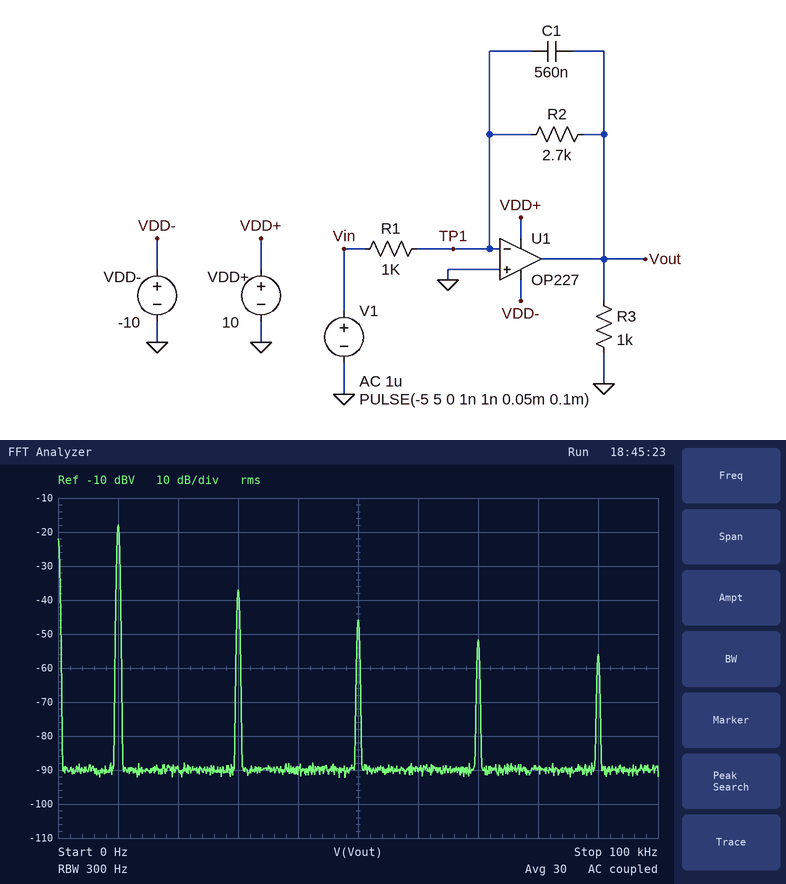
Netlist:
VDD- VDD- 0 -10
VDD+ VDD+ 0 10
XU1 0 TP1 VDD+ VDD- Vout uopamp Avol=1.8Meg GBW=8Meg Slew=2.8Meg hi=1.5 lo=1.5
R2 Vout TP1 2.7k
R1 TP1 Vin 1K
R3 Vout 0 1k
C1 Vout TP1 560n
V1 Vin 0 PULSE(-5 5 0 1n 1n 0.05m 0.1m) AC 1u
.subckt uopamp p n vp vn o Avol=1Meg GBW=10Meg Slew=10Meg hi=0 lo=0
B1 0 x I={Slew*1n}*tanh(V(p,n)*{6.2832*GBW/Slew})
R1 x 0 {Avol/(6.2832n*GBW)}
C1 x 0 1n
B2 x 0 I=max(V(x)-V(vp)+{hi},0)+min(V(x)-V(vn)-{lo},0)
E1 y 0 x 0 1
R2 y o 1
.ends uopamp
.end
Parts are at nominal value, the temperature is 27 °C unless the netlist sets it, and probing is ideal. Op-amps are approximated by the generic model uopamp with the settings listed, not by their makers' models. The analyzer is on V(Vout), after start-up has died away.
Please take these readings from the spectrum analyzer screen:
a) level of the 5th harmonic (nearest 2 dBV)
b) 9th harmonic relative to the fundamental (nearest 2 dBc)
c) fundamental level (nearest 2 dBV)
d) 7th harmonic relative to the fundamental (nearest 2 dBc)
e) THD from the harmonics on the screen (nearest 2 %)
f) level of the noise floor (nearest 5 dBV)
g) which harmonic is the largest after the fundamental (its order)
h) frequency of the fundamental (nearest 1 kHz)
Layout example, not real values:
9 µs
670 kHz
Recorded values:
-46 dBV
-38 dBc
-18 dBV
-34 dBc
12 %
-90 dBV
3
10 kHz
